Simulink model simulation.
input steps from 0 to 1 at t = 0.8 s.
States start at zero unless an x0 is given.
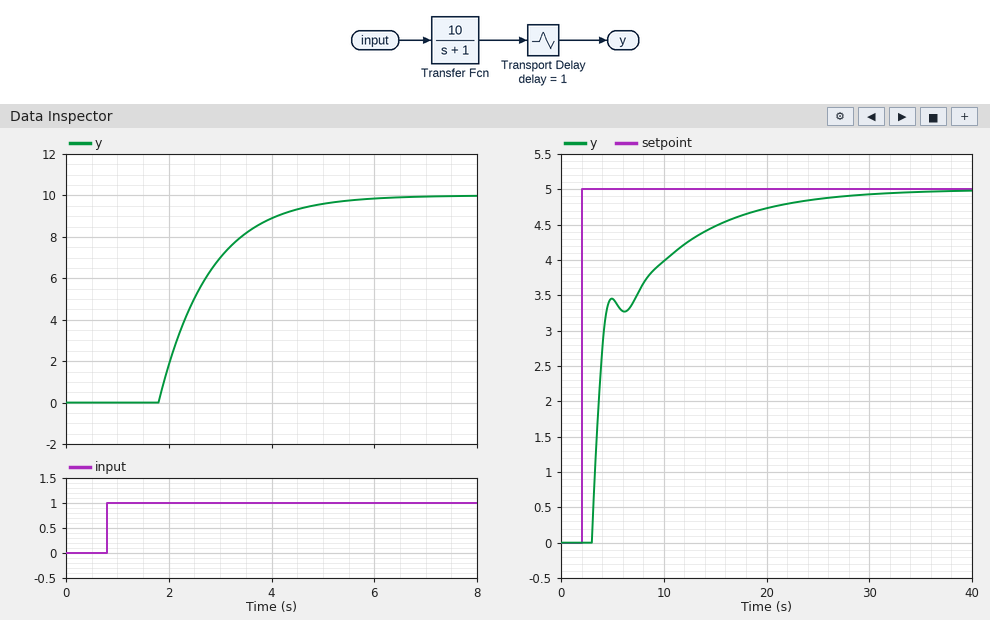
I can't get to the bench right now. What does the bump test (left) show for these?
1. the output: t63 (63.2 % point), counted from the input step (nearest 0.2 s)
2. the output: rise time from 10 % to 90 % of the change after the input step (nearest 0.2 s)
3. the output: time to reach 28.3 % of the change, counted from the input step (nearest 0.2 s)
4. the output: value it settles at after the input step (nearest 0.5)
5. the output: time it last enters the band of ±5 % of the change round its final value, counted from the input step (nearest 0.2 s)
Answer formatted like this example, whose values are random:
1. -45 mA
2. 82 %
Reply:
1. 2.0 s
2. 2.2 s
3. 1.4 s
4. 10.0
5. 4.0 s
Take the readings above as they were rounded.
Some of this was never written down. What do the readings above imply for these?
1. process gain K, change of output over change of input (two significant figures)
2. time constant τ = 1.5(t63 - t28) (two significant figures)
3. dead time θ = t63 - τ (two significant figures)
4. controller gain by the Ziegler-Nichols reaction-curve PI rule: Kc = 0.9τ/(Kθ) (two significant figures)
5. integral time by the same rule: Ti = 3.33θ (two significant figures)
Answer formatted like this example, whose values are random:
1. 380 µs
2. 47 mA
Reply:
1. 10
2. 0.90 s
3. 1.1 s
4. 0.074
5. 3.7 s
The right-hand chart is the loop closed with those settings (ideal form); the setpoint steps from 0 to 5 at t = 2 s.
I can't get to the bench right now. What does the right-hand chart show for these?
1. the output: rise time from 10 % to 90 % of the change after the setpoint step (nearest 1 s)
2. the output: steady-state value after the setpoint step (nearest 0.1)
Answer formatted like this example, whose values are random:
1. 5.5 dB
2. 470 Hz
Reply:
1. 12 s
2. 5.0
